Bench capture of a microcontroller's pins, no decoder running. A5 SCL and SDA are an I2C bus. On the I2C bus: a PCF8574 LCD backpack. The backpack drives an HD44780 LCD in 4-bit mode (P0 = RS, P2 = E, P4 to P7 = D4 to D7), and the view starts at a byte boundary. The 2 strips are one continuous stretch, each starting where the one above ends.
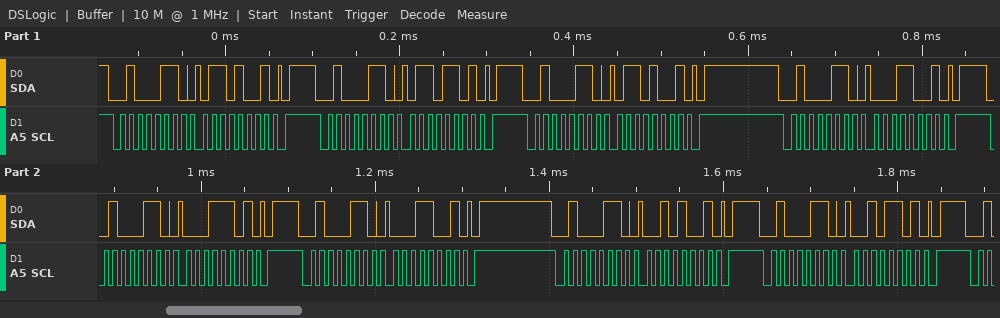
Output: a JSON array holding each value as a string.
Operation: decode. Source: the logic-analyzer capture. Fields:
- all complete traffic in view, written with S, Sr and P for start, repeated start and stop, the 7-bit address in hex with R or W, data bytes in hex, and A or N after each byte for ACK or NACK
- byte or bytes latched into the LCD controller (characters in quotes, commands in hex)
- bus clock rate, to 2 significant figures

["S 23W A 69 A P S 23W A 6D A P S 23W A 69 A P S 23W A 19 A P S 23W A 1D A P S 23W A 19 A P S 23W A 29 A P S 23W A 2D A P", "'a'", "100 kHz"]
